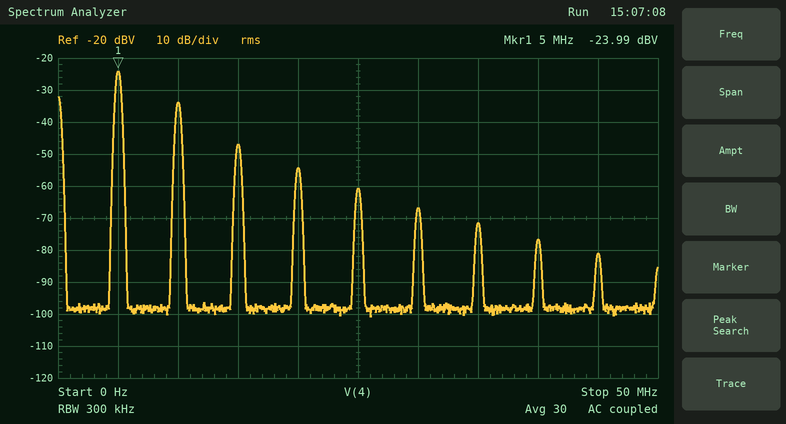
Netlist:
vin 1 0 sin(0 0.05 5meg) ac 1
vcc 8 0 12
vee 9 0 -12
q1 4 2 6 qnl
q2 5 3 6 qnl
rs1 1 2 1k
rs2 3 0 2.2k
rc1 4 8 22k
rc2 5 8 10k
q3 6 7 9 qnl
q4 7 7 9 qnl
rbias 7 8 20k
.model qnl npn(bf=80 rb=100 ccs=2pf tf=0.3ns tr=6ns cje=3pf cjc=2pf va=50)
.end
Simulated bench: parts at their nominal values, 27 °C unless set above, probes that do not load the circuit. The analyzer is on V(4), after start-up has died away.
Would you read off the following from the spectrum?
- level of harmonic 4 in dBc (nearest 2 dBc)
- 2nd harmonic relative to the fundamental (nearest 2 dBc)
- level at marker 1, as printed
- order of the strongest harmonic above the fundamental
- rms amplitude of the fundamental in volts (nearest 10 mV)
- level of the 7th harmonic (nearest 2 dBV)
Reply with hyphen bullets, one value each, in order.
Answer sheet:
- -30 dBc
- -10 dBc
- -23.99 dBV
- 2
- 60 mV
- -72 dBV
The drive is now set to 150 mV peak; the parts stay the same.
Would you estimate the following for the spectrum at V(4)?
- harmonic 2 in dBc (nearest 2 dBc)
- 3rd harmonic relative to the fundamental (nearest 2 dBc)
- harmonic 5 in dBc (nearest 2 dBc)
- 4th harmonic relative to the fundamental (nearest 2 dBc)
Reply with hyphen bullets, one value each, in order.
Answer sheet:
- -14 dBc
- -26 dBc
- -38 dBc
- -36 dBc
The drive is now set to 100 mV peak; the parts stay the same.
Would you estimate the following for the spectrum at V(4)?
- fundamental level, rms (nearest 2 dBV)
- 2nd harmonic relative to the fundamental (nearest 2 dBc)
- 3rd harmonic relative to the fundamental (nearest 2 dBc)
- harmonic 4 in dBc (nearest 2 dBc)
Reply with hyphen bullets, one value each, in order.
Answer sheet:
- -12 dBV
- -12 dBc
- -26 dBc
- -32 dBc
